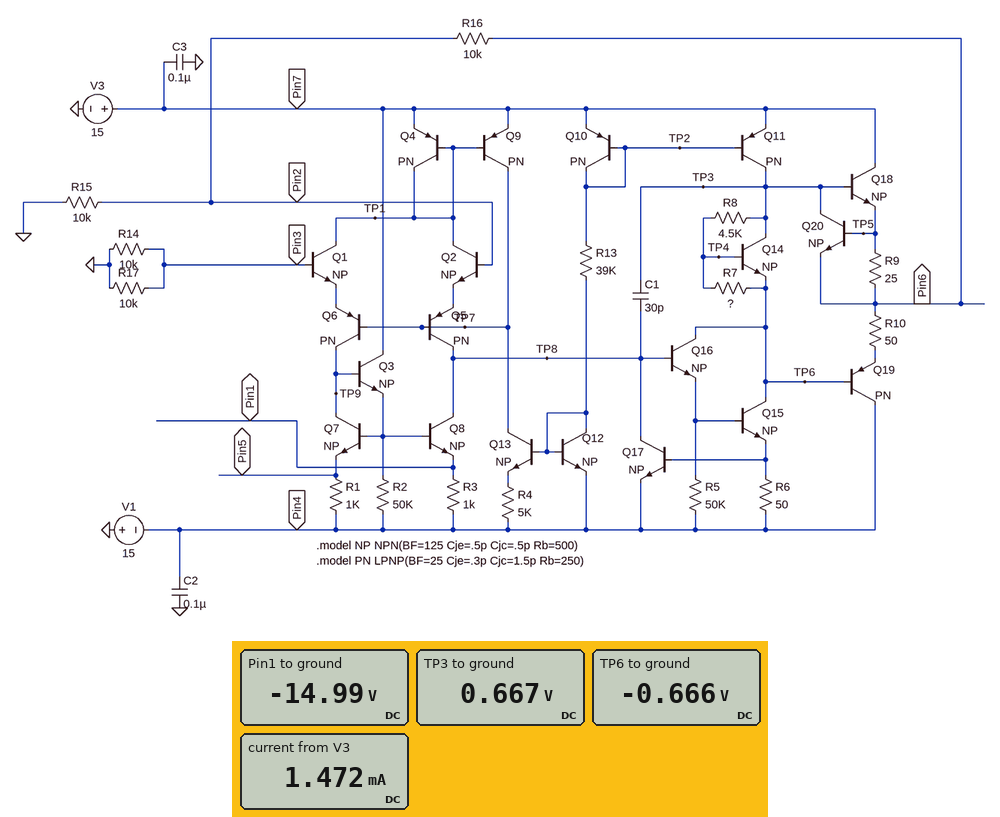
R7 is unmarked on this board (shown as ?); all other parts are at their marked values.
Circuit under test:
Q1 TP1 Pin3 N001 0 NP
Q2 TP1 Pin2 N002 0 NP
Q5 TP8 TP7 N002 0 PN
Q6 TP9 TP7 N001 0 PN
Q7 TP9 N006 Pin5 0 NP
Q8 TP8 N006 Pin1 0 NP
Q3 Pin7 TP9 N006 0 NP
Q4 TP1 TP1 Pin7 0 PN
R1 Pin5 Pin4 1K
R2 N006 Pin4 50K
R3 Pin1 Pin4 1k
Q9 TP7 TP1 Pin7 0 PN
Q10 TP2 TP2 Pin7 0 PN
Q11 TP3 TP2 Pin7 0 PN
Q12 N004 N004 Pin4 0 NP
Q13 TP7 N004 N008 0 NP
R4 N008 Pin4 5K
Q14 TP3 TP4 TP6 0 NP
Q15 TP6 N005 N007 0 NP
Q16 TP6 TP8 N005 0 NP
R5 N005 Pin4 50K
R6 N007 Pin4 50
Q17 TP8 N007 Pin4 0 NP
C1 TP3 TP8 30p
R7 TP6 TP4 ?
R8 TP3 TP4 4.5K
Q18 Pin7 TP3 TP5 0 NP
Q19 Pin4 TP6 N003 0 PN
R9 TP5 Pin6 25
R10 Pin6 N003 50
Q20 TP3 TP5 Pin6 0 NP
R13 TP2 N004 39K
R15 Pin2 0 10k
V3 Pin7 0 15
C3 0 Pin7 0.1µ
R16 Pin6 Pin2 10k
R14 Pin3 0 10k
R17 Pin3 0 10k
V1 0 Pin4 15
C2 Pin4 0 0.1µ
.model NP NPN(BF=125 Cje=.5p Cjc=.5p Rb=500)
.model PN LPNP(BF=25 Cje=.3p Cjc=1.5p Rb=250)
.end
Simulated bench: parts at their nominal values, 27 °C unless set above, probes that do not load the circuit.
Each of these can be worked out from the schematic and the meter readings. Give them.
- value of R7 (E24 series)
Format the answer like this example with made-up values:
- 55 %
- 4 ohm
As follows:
- 6.2 kΩ
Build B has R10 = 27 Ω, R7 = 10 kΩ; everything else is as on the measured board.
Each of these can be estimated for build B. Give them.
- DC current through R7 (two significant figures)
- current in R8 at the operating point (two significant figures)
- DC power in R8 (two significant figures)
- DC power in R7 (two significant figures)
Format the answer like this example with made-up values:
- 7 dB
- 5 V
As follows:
- 76 µA
- 81 µA
- 30 µW
- 58 µW
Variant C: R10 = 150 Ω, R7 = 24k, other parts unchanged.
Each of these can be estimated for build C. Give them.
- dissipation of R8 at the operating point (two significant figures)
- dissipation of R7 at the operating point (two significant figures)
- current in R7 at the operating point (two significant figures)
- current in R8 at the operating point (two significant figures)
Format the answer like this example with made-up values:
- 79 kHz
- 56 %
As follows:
- 6.2 µW
- 24 µW
- 32 µA
- 37 µA
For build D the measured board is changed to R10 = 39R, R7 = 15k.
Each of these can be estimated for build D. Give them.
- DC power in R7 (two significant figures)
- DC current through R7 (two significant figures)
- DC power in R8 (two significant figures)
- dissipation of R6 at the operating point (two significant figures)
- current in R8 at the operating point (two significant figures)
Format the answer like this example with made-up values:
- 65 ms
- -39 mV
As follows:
- 39 µW
- 51 µA
- 14 µW
- 22 µW
- 56 µA
